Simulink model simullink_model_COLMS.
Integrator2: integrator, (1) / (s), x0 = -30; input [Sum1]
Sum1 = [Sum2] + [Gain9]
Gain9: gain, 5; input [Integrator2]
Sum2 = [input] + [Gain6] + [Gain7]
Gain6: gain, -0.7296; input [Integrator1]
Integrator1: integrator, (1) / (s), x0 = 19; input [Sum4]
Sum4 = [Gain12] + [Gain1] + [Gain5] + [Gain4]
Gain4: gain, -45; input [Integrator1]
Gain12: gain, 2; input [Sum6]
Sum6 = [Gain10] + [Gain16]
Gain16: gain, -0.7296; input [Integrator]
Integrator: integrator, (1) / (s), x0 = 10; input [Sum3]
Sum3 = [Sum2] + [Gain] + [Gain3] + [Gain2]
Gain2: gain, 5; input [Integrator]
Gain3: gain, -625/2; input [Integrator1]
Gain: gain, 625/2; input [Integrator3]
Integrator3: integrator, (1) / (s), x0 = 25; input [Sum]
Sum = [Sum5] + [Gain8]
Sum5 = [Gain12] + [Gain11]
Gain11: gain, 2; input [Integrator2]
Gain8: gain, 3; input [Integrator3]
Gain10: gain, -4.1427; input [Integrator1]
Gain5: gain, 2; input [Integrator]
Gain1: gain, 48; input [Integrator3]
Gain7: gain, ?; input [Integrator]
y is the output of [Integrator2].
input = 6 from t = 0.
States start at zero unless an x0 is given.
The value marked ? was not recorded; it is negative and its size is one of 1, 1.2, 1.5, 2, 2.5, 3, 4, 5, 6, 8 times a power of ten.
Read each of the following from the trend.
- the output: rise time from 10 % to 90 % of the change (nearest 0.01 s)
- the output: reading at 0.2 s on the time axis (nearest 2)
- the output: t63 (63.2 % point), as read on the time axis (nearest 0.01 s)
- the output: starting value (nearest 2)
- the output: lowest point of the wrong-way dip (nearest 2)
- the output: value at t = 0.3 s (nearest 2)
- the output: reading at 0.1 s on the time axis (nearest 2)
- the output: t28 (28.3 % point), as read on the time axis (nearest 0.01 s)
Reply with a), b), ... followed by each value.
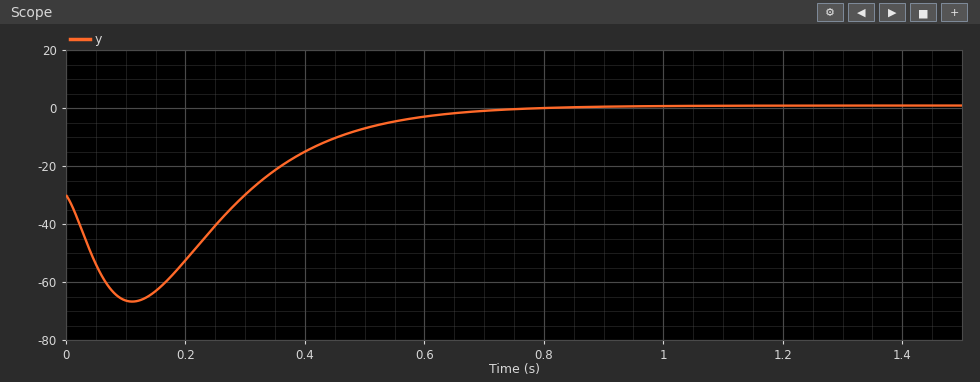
a) 0.31 s
b) -52
c) 0.45 s
d) -30
e) -66
f) -30
g) -66
h) 0.35 s
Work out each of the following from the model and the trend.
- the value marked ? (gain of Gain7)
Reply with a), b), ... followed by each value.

a) -12
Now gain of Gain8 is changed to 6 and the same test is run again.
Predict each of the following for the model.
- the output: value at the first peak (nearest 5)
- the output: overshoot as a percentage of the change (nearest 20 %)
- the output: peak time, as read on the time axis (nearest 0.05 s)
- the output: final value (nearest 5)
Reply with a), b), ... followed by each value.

a) 15
b) 40 %
c) 0.60 s
d) 0
